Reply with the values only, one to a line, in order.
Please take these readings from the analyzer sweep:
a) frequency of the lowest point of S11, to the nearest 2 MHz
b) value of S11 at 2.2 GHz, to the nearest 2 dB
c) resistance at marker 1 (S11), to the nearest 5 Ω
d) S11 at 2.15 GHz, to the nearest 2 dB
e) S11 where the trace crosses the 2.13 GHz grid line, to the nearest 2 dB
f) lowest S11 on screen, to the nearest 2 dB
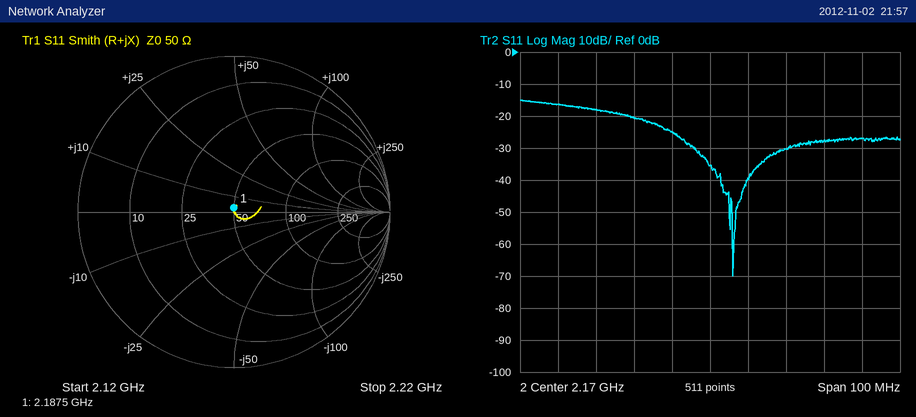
2.176 GHz
-28 dB
50 Ω
-20 dB
-16 dB
-70 dB
